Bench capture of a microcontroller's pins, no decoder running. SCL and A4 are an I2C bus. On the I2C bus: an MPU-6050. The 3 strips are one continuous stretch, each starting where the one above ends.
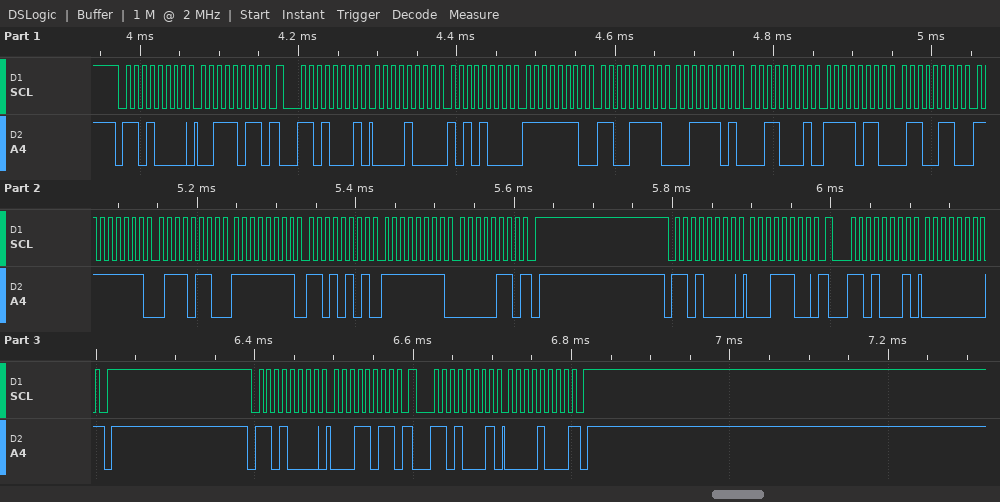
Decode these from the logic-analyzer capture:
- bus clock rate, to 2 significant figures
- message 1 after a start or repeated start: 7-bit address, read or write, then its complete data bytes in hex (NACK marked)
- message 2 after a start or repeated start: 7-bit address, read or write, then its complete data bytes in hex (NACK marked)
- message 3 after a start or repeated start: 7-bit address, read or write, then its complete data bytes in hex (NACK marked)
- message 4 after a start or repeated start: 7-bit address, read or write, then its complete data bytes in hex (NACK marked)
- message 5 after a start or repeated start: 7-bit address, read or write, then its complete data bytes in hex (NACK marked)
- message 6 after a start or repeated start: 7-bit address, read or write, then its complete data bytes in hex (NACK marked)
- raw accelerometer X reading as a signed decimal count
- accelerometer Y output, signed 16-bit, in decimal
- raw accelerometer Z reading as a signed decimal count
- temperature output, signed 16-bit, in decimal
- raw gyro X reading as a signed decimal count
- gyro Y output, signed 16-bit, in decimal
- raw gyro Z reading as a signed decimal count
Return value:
100 kHz
0x68 write: 3B
0x68 read: 08 A8 FE CF 3D 31 F6 66 FF 76 FF D5 FF 06 NACK
0x68 write: 1C
0x68 read: 00 NACK
0x68 write: 1B
0x68 read: 08 NACK
2216
-305
15665
-2458
-138
-43
-250
